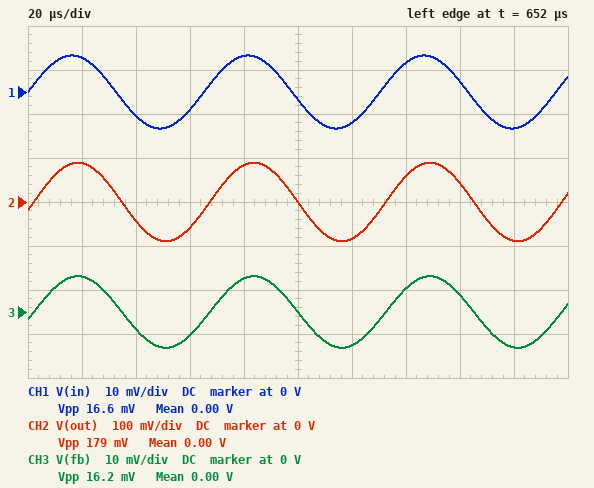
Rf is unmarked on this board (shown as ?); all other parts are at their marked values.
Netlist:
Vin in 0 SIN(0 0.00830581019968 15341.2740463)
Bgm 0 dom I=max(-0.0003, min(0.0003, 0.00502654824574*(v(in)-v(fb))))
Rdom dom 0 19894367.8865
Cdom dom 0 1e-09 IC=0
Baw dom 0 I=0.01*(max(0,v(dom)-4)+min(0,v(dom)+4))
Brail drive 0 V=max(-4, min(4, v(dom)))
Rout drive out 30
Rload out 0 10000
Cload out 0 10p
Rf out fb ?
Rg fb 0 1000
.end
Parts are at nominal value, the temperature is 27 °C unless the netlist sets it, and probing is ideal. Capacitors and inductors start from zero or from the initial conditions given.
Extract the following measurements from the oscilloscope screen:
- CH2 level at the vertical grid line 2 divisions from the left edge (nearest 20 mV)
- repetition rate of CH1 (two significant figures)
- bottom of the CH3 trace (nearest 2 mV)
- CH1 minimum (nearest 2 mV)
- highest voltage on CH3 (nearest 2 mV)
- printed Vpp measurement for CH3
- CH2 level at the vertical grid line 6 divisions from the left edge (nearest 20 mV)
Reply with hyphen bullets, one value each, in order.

- -40 mV
- 15 kHz
- -8 mV
- -8 mV
- 8 mV
- 16.2 mV
- -80 mV
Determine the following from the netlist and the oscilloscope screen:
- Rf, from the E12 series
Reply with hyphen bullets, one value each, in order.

- 10 kΩ
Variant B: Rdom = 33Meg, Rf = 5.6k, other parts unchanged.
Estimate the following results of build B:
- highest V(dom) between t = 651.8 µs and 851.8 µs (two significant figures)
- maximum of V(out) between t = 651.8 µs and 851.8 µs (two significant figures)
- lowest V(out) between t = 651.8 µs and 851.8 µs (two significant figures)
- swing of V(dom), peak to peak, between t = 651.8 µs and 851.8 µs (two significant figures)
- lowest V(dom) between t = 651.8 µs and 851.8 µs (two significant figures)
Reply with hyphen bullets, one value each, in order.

- 55 mV
- 54 mV
- -54 mV
- 110 mV
- -55 mV
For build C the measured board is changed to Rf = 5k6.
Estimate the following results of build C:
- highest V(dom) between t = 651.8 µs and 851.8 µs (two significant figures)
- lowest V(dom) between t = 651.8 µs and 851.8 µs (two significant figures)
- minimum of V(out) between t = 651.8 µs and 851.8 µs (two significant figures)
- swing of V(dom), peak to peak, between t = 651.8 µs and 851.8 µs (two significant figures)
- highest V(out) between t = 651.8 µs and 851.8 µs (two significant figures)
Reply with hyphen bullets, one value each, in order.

- 55 mV
- -55 mV
- -54 mV
- 110 mV
- 54 mV
